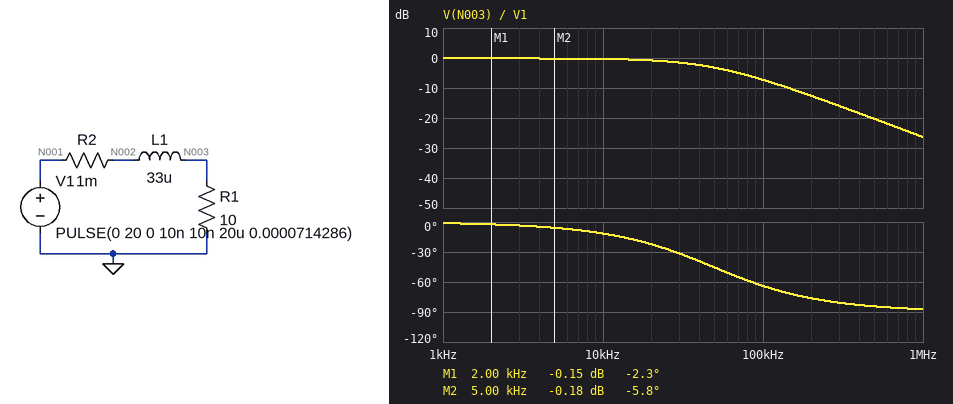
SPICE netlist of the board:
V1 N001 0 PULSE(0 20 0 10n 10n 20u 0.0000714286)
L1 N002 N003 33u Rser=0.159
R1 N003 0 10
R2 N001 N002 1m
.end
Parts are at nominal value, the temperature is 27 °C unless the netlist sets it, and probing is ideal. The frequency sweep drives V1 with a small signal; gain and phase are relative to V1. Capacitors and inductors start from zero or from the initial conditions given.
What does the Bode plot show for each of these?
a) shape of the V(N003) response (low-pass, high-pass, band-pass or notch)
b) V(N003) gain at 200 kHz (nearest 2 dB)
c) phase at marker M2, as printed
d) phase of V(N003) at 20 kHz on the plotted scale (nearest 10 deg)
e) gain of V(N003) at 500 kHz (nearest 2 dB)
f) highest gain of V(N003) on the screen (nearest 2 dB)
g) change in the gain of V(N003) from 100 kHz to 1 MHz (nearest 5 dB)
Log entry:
low-pass
-12 dB
-5.8 deg
-20 deg
-20 dB
0 dB
-20 dB
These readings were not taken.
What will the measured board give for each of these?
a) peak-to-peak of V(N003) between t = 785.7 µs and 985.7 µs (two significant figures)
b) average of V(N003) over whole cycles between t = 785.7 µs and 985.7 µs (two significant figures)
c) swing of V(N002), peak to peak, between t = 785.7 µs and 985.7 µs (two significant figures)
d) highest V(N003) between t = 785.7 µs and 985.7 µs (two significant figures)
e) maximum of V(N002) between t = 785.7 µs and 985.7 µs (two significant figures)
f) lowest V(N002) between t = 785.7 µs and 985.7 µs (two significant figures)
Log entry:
20 V
5.5 V
20 V
20 V
20 V
-2.0 mV
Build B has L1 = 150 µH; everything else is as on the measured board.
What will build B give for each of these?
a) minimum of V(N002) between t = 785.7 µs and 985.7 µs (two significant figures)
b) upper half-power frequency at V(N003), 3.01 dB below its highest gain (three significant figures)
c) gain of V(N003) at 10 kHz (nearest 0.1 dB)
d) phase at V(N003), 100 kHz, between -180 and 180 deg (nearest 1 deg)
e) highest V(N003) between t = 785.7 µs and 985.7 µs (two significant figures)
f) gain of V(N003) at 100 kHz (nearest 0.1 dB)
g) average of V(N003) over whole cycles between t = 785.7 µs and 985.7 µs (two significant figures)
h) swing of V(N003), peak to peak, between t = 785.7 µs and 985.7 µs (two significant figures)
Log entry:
-1.5 mV
10.8 kHz
-2.8 dB
-84 deg
15 V
-19.5 dB
5.5 V
14 V
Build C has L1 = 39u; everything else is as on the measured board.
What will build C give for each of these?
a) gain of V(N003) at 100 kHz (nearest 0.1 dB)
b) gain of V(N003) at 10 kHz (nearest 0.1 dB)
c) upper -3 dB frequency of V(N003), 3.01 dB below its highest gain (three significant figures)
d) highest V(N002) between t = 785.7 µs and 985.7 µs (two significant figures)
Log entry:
-8.5 dB
-0.4 dB
41.5 kHz
20 V
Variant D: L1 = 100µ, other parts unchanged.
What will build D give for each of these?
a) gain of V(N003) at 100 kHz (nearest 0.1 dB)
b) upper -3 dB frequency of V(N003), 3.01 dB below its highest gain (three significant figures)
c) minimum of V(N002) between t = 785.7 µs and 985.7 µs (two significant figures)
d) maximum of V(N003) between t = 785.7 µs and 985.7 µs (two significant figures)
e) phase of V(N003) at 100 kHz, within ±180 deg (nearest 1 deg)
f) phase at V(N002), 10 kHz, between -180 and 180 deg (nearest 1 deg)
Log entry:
-16.1 dB
16.2 kHz
-1.7 mV
17 V
-81 deg
0 deg
